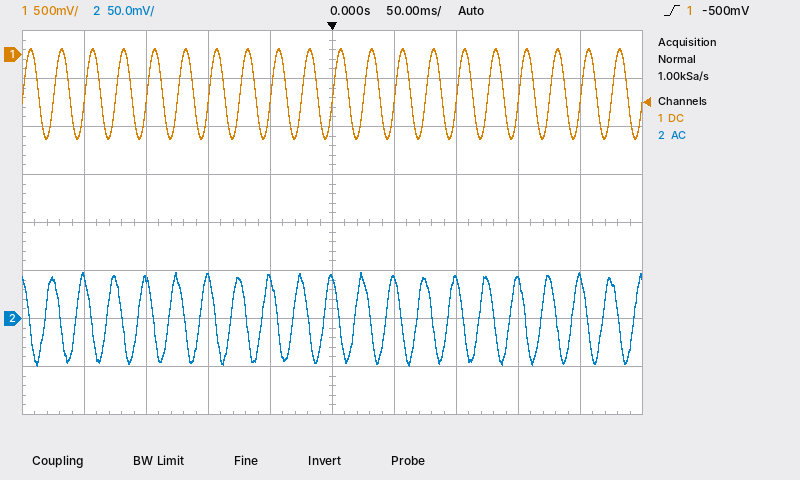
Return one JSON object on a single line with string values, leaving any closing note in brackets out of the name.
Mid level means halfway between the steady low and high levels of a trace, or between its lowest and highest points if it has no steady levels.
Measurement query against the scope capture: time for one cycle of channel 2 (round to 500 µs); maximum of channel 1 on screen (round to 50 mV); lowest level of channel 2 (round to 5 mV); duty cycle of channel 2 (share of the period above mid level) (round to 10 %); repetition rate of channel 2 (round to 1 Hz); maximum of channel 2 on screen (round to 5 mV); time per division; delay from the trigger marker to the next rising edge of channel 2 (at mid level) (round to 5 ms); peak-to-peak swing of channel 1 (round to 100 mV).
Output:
{"time for one cycle of channel 2": "25.0 ms", "maximum of channel 1 on screen": "50 mV", "lowest level of channel 2": "-50 mV", "duty cycle of channel 2 (share of the period above mid level)": "50 %", "repetition rate of channel 2": "40 Hz", "maximum of channel 2 on screen": "50 mV", "time per division": "50 ms", "delay from the trigger marker to the next rising edge of channel 2 (at mid level)": "20 ms", "peak-to-peak swing of channel 1": "900 mV"}
